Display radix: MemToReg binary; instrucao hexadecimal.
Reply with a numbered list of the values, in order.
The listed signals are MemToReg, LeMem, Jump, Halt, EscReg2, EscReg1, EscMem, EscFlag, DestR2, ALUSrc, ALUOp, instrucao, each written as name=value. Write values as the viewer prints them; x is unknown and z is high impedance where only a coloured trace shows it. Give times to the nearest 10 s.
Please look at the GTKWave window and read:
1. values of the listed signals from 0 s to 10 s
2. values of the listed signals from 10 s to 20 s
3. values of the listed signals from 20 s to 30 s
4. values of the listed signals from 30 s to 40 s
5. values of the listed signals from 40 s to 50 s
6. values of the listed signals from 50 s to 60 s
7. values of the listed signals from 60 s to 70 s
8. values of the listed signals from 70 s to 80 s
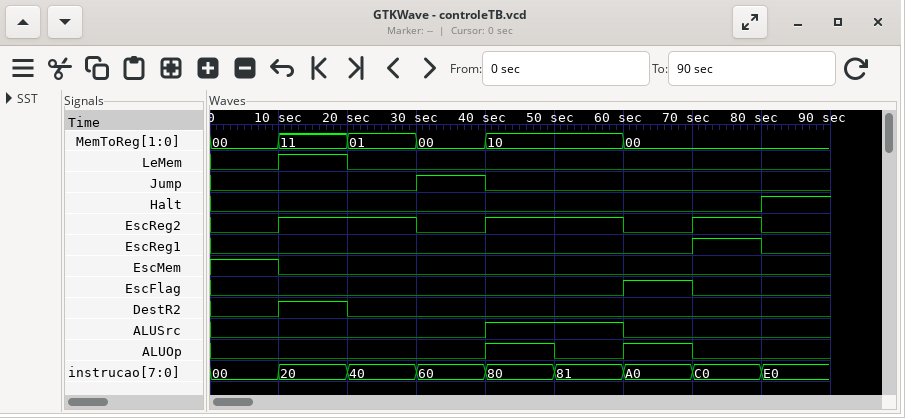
1. MemToReg=00, LeMem=0, Jump=0, Halt=0, EscReg2=0, EscReg1=0, EscMem=1, EscFlag=0, DestR2=0, ALUSrc=0, ALUOp=0, instrucao=00
2. MemToReg=11, LeMem=1, Jump=0, Halt=0, EscReg2=1, EscReg1=0, EscMem=0, EscFlag=0, DestR2=1, ALUSrc=0, ALUOp=0, instrucao=20
3. MemToReg=01, LeMem=0, Jump=0, Halt=0, EscReg2=1, EscReg1=0, EscMem=0, EscFlag=0, DestR2=0, ALUSrc=0, ALUOp=0, instrucao=40
4. MemToReg=00, LeMem=0, Jump=1, Halt=0, EscReg2=0, EscReg1=0, EscMem=0, EscFlag=0, DestR2=0, ALUSrc=0, ALUOp=0, instrucao=60
5. MemToReg=10, LeMem=0, Jump=0, Halt=0, EscReg2=1, EscReg1=0, EscMem=0, EscFlag=0, DestR2=0, ALUSrc=1, ALUOp=1, instrucao=80
6. MemToReg=10, LeMem=0, Jump=0, Halt=0, EscReg2=1, EscReg1=0, EscMem=0, EscFlag=0, DestR2=0, ALUSrc=1, ALUOp=0, instrucao=81
7. MemToReg=00, LeMem=0, Jump=0, Halt=0, EscReg2=0, EscReg1=0, EscMem=0, EscFlag=1, DestR2=0, ALUSrc=0, ALUOp=1, instrucao=A0
8. MemToReg=00, LeMem=0, Jump=0, Halt=0, EscReg2=1, EscReg1=1, EscMem=0, EscFlag=0, DestR2=0, ALUSrc=0, ALUOp=0, instrucao=C0
